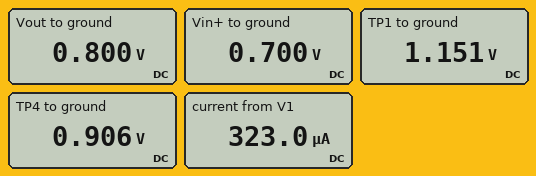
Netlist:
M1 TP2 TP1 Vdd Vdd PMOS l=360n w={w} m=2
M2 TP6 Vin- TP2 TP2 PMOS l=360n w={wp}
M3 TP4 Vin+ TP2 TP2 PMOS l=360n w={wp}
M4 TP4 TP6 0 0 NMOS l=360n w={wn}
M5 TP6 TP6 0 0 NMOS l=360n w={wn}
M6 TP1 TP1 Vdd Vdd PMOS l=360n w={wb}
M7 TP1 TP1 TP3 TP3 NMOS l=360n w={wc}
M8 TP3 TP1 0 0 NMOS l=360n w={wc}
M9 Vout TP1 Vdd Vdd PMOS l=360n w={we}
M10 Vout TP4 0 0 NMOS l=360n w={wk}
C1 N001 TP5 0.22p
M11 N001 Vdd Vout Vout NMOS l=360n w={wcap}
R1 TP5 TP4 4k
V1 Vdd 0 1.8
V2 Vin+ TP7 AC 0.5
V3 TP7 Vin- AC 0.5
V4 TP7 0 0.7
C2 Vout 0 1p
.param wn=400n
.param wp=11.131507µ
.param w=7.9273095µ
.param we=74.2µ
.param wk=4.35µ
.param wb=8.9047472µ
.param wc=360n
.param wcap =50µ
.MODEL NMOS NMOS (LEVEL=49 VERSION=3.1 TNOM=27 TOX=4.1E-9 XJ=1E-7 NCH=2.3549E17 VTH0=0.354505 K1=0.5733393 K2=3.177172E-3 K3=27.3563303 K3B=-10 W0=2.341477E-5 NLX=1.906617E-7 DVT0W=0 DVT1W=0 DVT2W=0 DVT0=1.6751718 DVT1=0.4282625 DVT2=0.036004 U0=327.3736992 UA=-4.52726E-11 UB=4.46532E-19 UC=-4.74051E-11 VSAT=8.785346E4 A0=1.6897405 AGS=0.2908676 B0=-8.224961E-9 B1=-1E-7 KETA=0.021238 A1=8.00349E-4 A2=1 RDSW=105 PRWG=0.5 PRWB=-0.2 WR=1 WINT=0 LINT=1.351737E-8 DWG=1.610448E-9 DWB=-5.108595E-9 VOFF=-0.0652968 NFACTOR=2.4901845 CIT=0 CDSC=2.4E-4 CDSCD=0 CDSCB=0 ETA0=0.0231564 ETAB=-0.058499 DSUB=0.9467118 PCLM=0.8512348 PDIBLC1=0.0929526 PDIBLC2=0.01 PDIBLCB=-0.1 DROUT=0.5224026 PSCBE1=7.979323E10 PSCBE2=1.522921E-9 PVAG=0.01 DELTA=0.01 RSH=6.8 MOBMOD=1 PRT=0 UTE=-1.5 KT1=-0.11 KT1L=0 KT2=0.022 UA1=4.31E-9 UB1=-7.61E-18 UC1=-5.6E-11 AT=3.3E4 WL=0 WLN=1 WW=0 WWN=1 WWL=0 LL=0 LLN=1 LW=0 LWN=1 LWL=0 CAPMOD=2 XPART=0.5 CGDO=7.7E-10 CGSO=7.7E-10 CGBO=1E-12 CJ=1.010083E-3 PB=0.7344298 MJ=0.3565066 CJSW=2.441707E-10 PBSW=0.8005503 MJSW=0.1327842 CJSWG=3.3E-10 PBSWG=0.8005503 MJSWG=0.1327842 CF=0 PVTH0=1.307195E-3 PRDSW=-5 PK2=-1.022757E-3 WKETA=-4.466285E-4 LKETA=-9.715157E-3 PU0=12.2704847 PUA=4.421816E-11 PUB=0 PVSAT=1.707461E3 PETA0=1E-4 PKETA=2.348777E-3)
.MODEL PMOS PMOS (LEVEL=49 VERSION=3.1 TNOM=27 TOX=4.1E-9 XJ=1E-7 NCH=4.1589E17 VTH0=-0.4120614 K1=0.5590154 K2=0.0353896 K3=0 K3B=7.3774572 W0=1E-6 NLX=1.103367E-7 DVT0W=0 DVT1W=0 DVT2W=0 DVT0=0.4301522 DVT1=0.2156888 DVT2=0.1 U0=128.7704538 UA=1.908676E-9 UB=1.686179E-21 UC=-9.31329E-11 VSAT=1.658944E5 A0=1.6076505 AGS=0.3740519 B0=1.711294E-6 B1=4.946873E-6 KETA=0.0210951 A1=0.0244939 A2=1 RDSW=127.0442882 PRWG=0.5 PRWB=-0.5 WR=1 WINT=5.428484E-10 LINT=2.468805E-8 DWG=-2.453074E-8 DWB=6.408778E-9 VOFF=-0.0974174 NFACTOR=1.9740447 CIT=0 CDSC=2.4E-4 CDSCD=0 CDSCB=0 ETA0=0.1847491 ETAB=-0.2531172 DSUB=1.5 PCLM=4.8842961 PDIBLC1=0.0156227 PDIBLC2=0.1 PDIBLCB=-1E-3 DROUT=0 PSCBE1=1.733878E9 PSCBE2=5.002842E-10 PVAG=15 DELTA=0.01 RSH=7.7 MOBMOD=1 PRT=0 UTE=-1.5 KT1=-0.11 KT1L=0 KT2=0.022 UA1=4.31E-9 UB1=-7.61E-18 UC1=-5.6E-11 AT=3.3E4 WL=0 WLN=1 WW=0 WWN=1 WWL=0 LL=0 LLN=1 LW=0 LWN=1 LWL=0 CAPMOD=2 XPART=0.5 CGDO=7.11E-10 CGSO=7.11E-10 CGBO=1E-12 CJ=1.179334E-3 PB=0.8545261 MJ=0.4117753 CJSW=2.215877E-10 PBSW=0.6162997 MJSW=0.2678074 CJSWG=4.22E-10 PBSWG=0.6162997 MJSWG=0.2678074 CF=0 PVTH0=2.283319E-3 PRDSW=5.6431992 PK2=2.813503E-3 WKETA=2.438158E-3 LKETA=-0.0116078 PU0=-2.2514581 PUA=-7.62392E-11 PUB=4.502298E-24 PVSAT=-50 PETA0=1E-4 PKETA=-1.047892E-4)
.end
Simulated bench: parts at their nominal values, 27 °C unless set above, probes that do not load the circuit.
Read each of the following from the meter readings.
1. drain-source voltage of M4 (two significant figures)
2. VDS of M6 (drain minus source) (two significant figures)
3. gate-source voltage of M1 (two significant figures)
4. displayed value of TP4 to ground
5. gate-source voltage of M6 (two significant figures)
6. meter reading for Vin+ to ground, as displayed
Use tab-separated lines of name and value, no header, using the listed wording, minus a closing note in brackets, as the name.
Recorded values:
drain-source voltage of M4	910 mV
VDS of M6 (drain minus source)	-650 mV
gate-source voltage of M1	-650 mV
displayed value of TP4 to ground	0.906 V
gate-source voltage of M6	-650 mV
meter reading for Vin+ to ground, as displayed	0.700 V
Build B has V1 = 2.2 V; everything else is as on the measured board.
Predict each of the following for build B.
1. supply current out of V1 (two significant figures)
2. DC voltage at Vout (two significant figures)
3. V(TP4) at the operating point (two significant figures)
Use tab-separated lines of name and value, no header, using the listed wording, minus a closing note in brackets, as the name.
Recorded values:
supply current out of V1	640 µA
DC voltage at Vout	880 mV
V(TP4) at the operating point	1.1 V
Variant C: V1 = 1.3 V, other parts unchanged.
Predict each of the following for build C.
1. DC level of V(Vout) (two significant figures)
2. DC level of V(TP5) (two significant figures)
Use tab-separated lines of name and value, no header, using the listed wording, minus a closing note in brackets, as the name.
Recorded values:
DC level of V(Vout)	710 mV
DC level of V(TP5)	660 mV
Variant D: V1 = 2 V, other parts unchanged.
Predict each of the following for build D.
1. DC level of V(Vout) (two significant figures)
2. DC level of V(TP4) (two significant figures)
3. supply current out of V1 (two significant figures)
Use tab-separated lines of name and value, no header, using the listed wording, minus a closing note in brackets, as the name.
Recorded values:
DC level of V(Vout)	850 mV
DC level of V(TP4)	1.0 V
supply current out of V1	470 µA
